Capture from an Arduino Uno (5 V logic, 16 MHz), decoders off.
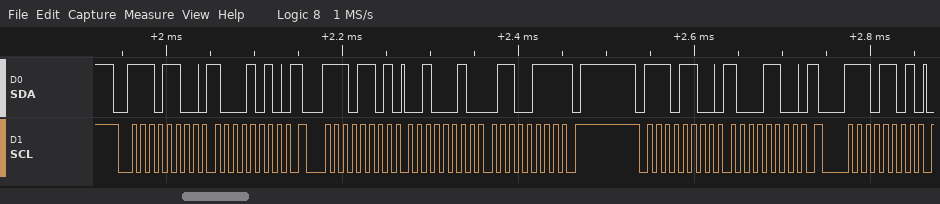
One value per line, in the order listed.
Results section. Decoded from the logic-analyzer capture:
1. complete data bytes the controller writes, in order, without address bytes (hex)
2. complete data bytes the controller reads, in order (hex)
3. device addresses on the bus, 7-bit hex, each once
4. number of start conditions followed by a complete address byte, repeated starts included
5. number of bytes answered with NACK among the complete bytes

8A 8C
22 67
0x76
4
1
